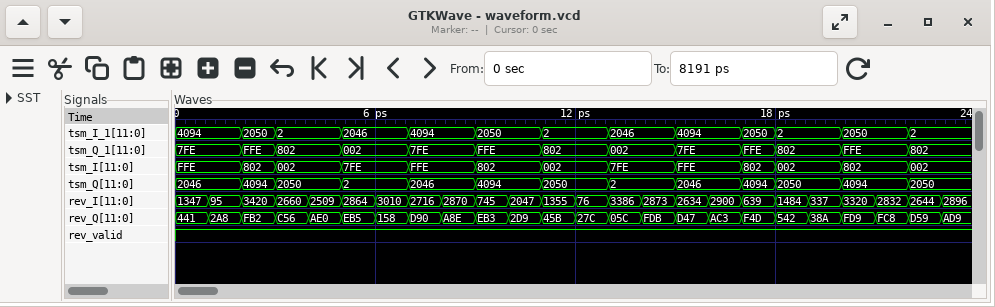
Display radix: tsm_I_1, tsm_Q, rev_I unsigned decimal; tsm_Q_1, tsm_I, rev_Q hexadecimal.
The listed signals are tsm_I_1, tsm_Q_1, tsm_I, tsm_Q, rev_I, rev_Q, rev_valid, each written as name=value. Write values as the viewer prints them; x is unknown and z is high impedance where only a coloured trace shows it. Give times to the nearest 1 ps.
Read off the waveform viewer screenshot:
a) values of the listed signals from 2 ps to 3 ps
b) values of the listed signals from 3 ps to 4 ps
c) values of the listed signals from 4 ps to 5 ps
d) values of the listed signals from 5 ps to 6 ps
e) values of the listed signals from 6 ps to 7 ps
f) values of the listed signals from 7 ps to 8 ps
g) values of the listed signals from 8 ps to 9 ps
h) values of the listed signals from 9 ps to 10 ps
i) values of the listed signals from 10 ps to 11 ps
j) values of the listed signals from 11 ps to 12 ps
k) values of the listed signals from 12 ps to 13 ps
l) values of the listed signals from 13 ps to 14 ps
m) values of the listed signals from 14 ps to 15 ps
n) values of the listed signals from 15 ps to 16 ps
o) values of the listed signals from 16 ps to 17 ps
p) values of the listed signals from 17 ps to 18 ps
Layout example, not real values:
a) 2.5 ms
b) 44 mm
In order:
a) tsm_I_1=2050, tsm_Q_1=FFE, tsm_I=802, tsm_Q=4094, rev_I=3420, rev_Q=FB2, rev_valid=1
b) tsm_I_1=2, tsm_Q_1=802, tsm_I=002, tsm_Q=2050, rev_I=2660, rev_Q=C56, rev_valid=1
c) tsm_I_1=2, tsm_Q_1=802, tsm_I=002, tsm_Q=2050, rev_I=2509, rev_Q=AE0, rev_valid=1
d) tsm_I_1=2046, tsm_Q_1=002, tsm_I=7FE, tsm_Q=2, rev_I=2864, rev_Q=EB5, rev_valid=1
e) tsm_I_1=2046, tsm_Q_1=002, tsm_I=7FE, tsm_Q=2, rev_I=3010, rev_Q=158, rev_valid=1
f) tsm_I_1=4094, tsm_Q_1=7FE, tsm_I=FFE, tsm_Q=2046, rev_I=2716, rev_Q=D90, rev_valid=1
g) tsm_I_1=4094, tsm_Q_1=7FE, tsm_I=FFE, tsm_Q=2046, rev_I=2870, rev_Q=A8E, rev_valid=1
h) tsm_I_1=2050, tsm_Q_1=FFE, tsm_I=802, tsm_Q=4094, rev_I=745, rev_Q=EB3, rev_valid=1
i) tsm_I_1=2050, tsm_Q_1=FFE, tsm_I=802, tsm_Q=4094, rev_I=2047, rev_Q=2D9, rev_valid=1
j) tsm_I_1=2, tsm_Q_1=802, tsm_I=002, tsm_Q=2050, rev_I=1355, rev_Q=45B, rev_valid=1
k) tsm_I_1=2, tsm_Q_1=802, tsm_I=002, tsm_Q=2050, rev_I=76, rev_Q=27C, rev_valid=1
l) tsm_I_1=2046, tsm_Q_1=002, tsm_I=7FE, tsm_Q=2, rev_I=3386, rev_Q=05C, rev_valid=1
m) tsm_I_1=2046, tsm_Q_1=002, tsm_I=7FE, tsm_Q=2, rev_I=2873, rev_Q=FDB, rev_valid=1
n) tsm_I_1=4094, tsm_Q_1=7FE, tsm_I=FFE, tsm_Q=2046, rev_I=2634, rev_Q=D47, rev_valid=1
o) tsm_I_1=4094, tsm_Q_1=7FE, tsm_I=FFE, tsm_Q=2046, rev_I=2900, rev_Q=AC3, rev_valid=1
p) tsm_I_1=2050, tsm_Q_1=FFE, tsm_I=802, tsm_Q=4094, rev_I=639, rev_Q=F4D, rev_valid=1
